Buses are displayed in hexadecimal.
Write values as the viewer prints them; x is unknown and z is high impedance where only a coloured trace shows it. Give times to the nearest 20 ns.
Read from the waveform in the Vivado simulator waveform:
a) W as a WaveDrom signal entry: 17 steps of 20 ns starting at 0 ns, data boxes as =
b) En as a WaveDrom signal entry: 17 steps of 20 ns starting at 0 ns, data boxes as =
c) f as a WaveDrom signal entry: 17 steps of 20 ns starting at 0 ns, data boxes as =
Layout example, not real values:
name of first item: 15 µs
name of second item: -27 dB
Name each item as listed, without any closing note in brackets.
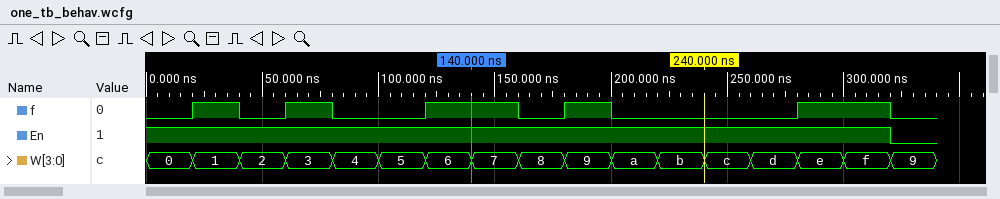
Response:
W as a WaveDrom signal entry: 17 steps of 20 ns starting at 0 ns, data boxes as =: {name: 'W', wave: '=================', data: '0 1 2 3 4 5 6 7 8 9 a b c d e f 9'}
En as a WaveDrom signal entry: 17 steps of 20 ns starting at 0 ns, data boxes as =: {name: 'En', wave: '1...............0'}
f as a WaveDrom signal entry: 17 steps of 20 ns starting at 0 ns, data boxes as =: {name: 'f', wave: '01010.1.010...1.0'}
